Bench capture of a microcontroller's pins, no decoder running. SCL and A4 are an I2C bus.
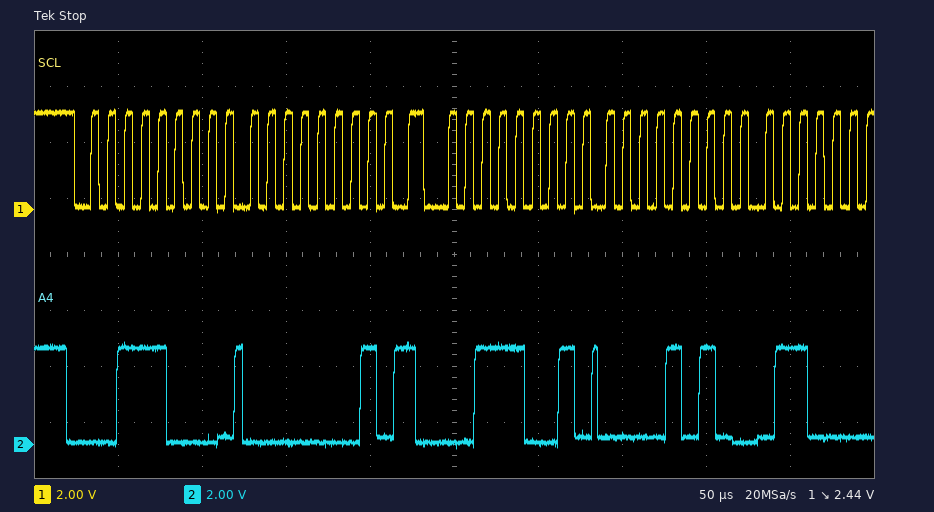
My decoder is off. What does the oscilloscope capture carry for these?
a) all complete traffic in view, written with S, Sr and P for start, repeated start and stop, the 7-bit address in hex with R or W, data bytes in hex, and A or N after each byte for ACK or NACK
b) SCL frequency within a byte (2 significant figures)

S 1CW A 01 A Sr 1CR A 0A A
100 kHz
